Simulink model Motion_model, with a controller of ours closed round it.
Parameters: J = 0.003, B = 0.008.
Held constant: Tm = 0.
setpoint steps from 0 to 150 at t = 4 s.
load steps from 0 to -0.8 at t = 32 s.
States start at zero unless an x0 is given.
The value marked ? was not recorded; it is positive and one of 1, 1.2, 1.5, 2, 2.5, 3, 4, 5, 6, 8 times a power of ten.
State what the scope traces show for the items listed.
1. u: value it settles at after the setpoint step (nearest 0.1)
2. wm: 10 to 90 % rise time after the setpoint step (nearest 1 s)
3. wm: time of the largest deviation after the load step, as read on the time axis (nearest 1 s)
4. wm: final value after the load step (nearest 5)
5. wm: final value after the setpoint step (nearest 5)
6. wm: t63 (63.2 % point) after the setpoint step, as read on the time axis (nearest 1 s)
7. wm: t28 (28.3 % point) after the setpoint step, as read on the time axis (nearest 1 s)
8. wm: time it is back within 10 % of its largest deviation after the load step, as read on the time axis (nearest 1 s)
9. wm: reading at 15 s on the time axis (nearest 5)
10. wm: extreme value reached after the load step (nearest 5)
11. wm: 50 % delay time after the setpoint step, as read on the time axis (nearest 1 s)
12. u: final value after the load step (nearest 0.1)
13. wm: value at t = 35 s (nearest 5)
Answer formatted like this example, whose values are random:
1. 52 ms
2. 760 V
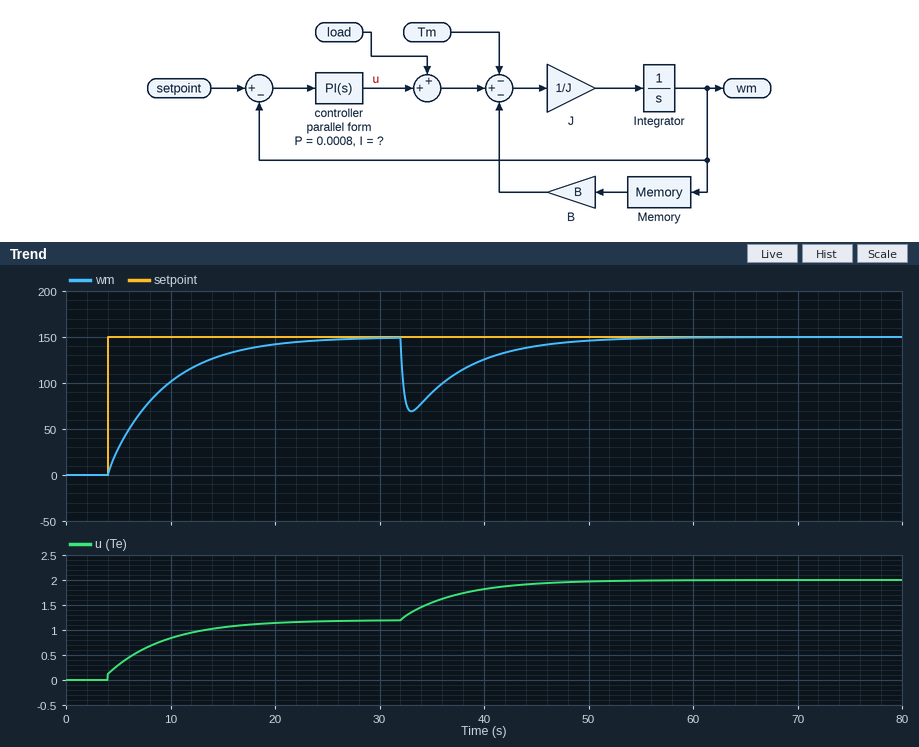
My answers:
1. 1.2
2. 12 s
3. 33 s
4. 150
5. 150
6. 9 s
7. 6 s
8. 46 s
9. 130
10. 70
11. 8 s
12. 2.0
13. 90
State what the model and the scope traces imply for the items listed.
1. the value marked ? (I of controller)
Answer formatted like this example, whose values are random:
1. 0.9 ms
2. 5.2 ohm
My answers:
1. 0.0015
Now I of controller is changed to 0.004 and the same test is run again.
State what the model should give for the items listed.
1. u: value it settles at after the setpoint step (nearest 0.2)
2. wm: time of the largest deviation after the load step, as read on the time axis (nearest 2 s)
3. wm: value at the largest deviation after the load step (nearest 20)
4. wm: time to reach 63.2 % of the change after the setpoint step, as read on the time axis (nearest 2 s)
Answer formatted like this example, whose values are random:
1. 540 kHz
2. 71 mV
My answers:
1. 1.2
2. 32 s
3. 80
4. 6 s
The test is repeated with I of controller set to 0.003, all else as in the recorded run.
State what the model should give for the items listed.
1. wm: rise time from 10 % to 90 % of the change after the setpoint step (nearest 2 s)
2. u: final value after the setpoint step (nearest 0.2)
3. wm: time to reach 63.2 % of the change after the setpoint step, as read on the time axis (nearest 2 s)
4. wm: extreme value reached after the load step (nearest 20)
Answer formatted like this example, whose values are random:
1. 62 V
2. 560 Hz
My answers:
1. 6 s
2. 1.2
3. 6 s
4. 80
